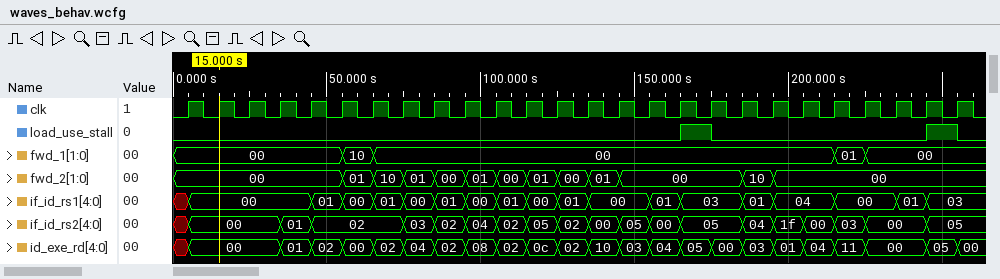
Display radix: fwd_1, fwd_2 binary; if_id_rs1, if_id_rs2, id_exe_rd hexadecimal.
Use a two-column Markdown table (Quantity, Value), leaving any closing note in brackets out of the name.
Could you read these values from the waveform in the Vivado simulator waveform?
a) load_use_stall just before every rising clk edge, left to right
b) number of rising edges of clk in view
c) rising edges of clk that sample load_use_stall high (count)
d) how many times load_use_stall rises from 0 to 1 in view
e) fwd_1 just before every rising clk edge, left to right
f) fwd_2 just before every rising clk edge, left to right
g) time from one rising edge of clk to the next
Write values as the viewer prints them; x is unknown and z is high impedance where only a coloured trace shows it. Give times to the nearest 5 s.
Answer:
| Quantity | Value |
|---|---|
| load_use_stall just before every rising clk edge, left to right | 0 0 0 0 0 0 0 0 0 0 0 0 0 0 0 0 0 1 0 0 0 0 0 0 0 1 |
| number of rising edges of clk in view | 26 |
| rising edges of clk that sample load_use_stall high | 2 |
| how many times load_use_stall rises from 0 to 1 in view | 2 |
| fwd_1 just before every rising clk edge, left to right | 00, 00, 00, 00, 00, 00, 10, 00, 00, 00, 00, 00, 00, 00, 00, 00, 00, 00, 00, 00, 00, 00, 01, 00, 00, 00 |
| fwd_2 just before every rising clk edge, left to right | 00, 00, 00, 00, 00, 00, 01, 10, 01, 00, 01, 00, 01, 00, 01, 00, 00, 00, 00, 10, 00, 00, 00, 00, 00, 00 |
| time from one rising edge of clk to the next | 10 s |
